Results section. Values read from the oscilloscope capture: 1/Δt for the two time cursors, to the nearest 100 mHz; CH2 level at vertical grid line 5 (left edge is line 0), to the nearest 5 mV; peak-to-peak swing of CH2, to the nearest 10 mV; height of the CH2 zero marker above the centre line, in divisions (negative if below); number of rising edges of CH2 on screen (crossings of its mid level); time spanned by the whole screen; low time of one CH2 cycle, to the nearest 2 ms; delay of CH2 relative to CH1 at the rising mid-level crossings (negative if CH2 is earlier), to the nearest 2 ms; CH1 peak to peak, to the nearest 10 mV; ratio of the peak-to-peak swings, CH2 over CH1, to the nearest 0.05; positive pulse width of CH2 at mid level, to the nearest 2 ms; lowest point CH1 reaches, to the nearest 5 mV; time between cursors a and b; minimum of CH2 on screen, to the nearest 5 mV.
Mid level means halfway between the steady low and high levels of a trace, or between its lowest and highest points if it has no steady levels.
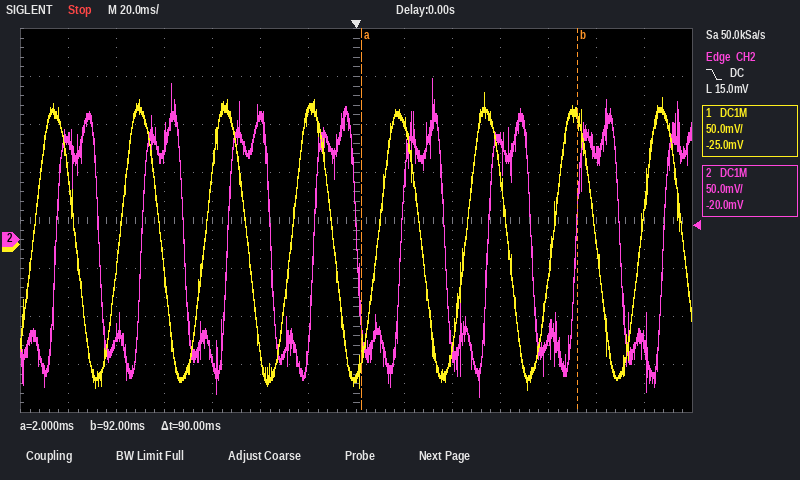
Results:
11.1 Hz
130 mV
330 mV
-0.4 div
8
280 ms
18 ms
+10 ms
310 mV
1.05
18 ms
-150 mV
90 ms
-165 mV
